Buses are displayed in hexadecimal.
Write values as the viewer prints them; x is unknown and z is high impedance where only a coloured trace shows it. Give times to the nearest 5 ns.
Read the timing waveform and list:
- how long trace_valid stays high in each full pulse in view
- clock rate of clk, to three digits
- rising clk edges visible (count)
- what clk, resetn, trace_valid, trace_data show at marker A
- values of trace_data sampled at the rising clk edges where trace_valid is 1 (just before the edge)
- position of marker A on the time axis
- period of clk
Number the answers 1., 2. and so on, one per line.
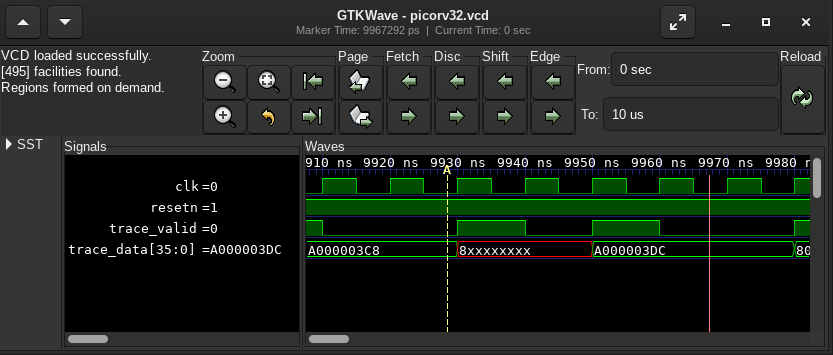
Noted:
1. 10 ns, 10 ns
2. 100 MHz
3. 8
4. clk=0, resetn=1, trace_valid=0, trace_data=A000003C8
5. A000003C8, 8xxxxxxxx, A000003DC
6. 9930 ns
7. 10 ns
